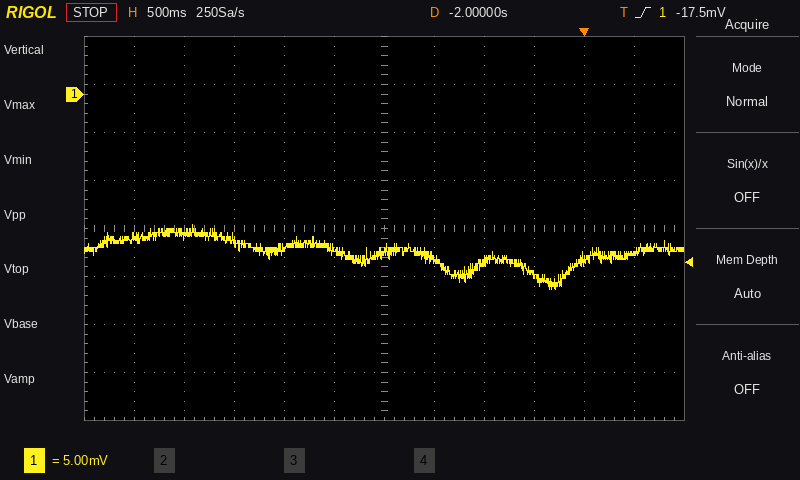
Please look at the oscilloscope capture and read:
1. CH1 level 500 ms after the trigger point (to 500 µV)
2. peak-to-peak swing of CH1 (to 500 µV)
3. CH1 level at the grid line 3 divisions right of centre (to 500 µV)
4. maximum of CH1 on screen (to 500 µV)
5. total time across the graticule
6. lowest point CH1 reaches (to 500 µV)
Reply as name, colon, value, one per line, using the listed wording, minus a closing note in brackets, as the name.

CH1 level 500 ms after the trigger point: -16.5 mV
peak-to-peak swing of CH1: 7.0 mV
CH1 level at the grid line 3 divisions right of centre: -19.0 mV
maximum of CH1 on screen: -13.5 mV
total time across the graticule: 6 s
lowest point CH1 reaches: -20.5 mV
